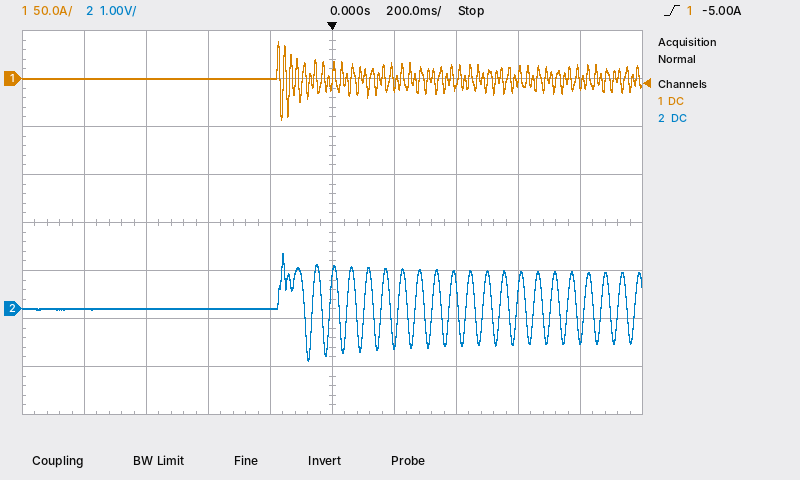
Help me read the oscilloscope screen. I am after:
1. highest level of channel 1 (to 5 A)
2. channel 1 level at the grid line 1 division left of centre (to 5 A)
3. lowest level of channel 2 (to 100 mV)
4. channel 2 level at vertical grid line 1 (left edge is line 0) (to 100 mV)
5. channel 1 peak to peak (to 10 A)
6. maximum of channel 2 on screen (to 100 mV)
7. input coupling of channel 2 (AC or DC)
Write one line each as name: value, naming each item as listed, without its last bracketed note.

highest level of channel 1: 40 A
channel 1 level at the grid line 1 division left of centre: 0 A
lowest level of channel 2: -1.1 V
channel 2 level at vertical grid line 1 (left edge is line 0): 0.0 V
channel 1 peak to peak: 80 A
maximum of channel 2 on screen: 1.2 V
input coupling of channel 2: DC
